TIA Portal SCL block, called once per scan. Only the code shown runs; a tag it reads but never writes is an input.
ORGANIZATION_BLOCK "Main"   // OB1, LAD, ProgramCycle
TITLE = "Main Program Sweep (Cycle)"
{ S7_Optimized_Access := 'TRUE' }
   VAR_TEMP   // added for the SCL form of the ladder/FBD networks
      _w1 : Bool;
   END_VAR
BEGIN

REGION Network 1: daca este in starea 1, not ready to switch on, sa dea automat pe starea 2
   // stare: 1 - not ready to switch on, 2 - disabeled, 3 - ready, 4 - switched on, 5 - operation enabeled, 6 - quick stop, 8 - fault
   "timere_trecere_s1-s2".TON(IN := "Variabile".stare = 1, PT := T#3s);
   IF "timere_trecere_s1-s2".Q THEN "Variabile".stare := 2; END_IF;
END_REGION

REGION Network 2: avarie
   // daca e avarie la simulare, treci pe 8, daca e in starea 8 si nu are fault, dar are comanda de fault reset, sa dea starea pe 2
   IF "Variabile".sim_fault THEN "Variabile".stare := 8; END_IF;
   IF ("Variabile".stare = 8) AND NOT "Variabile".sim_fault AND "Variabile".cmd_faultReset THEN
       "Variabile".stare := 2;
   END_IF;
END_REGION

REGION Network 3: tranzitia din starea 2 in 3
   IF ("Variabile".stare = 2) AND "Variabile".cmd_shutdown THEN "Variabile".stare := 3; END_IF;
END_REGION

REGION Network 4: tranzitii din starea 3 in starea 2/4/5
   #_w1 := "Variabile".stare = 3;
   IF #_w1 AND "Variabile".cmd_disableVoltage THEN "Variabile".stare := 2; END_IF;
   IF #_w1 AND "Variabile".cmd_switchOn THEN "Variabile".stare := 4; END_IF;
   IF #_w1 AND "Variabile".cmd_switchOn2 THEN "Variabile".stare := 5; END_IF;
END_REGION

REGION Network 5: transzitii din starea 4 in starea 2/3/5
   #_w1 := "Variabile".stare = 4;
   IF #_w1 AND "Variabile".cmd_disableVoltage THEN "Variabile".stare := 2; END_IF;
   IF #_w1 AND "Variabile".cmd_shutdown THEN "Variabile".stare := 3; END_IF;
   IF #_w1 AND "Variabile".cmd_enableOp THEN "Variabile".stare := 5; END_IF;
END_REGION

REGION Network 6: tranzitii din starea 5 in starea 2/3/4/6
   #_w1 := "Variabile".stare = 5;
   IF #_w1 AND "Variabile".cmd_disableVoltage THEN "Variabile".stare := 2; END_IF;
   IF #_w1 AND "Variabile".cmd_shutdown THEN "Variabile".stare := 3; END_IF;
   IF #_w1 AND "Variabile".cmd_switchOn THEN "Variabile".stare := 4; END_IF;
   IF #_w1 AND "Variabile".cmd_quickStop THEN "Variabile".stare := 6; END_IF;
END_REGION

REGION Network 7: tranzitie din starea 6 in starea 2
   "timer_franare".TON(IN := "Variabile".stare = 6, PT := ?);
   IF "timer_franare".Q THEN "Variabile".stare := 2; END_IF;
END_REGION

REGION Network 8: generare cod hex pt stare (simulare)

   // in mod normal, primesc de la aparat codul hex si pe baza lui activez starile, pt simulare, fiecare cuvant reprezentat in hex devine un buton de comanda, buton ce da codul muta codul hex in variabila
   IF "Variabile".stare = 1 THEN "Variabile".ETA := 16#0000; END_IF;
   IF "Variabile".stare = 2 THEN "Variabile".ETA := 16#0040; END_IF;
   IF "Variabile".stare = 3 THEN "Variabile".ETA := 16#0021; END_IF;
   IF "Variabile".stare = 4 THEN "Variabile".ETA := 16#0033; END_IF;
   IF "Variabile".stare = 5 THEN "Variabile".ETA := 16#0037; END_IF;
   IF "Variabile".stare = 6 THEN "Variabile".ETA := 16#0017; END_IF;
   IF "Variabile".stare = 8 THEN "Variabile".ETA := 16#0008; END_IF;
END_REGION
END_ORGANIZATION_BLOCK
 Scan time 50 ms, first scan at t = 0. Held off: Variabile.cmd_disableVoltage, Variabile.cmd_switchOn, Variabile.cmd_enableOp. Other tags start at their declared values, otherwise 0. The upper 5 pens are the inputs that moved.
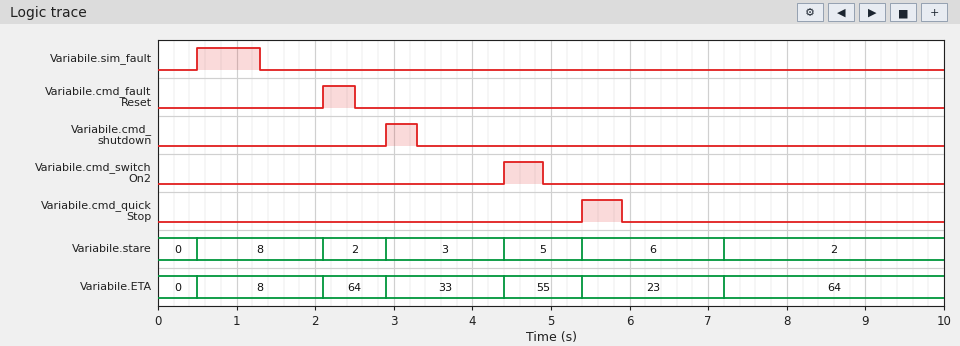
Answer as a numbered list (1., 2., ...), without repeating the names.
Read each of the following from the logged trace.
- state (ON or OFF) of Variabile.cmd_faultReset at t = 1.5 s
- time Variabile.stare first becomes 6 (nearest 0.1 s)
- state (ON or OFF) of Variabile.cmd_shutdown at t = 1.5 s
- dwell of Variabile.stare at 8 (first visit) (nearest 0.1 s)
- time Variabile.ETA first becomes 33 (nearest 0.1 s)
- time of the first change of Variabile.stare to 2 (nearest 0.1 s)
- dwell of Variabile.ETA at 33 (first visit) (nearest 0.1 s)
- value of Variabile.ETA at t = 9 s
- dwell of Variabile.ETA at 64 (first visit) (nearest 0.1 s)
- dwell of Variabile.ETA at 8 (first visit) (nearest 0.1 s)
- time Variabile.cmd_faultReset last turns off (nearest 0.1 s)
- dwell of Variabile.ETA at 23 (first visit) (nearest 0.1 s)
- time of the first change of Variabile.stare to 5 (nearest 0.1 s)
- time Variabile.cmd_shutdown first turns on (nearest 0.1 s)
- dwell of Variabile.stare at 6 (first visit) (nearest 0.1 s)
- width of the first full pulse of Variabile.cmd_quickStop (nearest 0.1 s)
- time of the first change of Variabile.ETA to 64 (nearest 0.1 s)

1. OFF
2. 5.4 s
3. OFF
4. 1.6 s
5. 2.9 s
6. 2.1 s
7. 1.5 s
8. 64
9. 0.8 s
10. 1.6 s
11. 2.5 s
12. 1.8 s
13. 4.4 s
14. 2.9 s
15. 1.8 s
16. 0.5 s
17. 2.1 s
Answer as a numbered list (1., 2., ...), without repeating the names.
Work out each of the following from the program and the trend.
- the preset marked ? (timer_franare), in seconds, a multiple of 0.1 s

1. 1.8 s
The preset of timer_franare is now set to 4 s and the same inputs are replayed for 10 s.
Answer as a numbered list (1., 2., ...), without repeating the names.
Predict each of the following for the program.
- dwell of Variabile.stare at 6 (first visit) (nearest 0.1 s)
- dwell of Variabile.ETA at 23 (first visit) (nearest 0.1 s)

1. 4.0 s
2. 4.0 s
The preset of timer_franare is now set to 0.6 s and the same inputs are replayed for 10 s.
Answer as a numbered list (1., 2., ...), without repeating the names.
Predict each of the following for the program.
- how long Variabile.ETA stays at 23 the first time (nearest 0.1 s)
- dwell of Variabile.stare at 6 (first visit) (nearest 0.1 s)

1. 0.6 s
2. 0.6 s
